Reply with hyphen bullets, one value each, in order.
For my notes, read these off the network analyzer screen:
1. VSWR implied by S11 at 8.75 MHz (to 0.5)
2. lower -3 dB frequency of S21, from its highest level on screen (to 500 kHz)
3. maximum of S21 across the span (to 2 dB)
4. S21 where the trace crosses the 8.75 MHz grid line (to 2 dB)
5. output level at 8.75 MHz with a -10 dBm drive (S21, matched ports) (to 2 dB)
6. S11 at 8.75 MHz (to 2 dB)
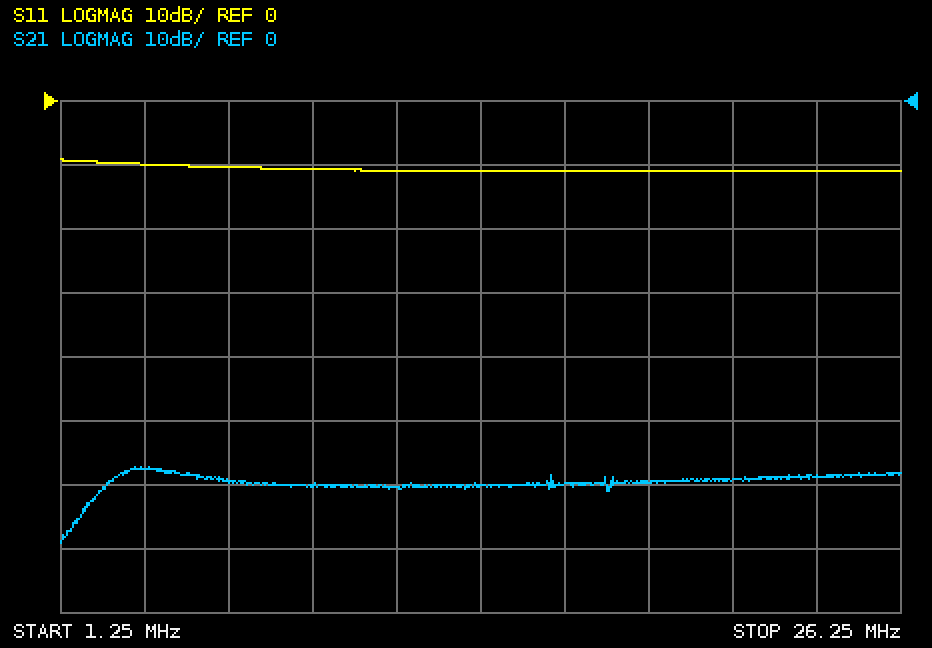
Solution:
- 2.0
- 2.5 MHz
- -58 dB
- -60 dB
- -70 dBm
- -10 dB
